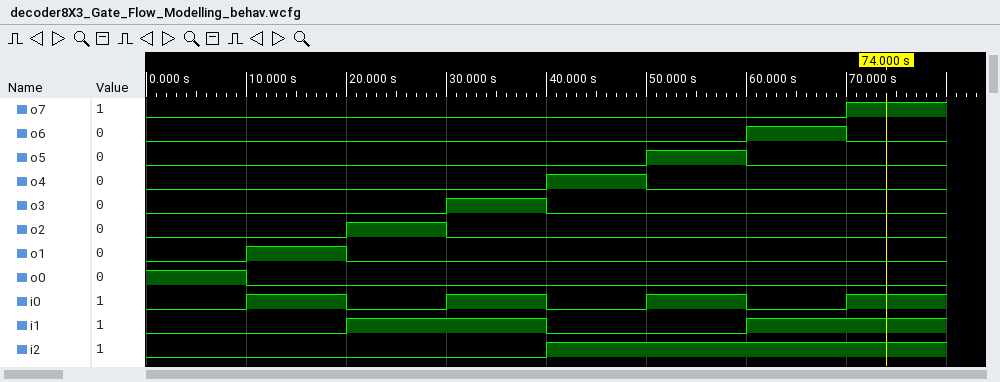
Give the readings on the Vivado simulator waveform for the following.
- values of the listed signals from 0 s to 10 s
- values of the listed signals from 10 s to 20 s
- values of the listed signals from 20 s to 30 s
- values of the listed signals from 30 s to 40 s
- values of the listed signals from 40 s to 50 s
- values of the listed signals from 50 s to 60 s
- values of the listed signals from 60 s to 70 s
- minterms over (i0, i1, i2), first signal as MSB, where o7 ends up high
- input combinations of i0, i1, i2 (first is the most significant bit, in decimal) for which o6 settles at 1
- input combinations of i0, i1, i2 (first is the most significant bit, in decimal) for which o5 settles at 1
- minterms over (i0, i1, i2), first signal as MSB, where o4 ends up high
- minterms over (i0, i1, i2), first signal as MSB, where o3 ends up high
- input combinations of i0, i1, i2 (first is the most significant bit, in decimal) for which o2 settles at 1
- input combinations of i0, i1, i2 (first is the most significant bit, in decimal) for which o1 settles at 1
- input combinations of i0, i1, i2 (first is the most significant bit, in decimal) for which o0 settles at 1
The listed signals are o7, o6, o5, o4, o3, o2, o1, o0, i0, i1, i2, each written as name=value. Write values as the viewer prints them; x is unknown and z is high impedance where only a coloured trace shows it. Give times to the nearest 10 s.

o7=0, o6=0, o5=0, o4=0, o3=0, o2=0, o1=0, o0=1, i0=0, i1=0, i2=0
o7=0, o6=0, o5=0, o4=0, o3=0, o2=0, o1=1, o0=0, i0=1, i1=0, i2=0
o7=0, o6=0, o5=0, o4=0, o3=0, o2=1, o1=0, o0=0, i0=0, i1=1, i2=0
o7=0, o6=0, o5=0, o4=0, o3=1, o2=0, o1=0, o0=0, i0=1, i1=1, i2=0
o7=0, o6=0, o5=0, o4=1, o3=0, o2=0, o1=0, o0=0, i0=0, i1=0, i2=1
o7=0, o6=0, o5=1, o4=0, o3=0, o2=0, o1=0, o0=0, i0=1, i1=0, i2=1
o7=0, o6=1, o5=0, o4=0, o3=0, o2=0, o1=0, o0=0, i0=0, i1=1, i2=1
7
3
5
1
6
2
4
0
